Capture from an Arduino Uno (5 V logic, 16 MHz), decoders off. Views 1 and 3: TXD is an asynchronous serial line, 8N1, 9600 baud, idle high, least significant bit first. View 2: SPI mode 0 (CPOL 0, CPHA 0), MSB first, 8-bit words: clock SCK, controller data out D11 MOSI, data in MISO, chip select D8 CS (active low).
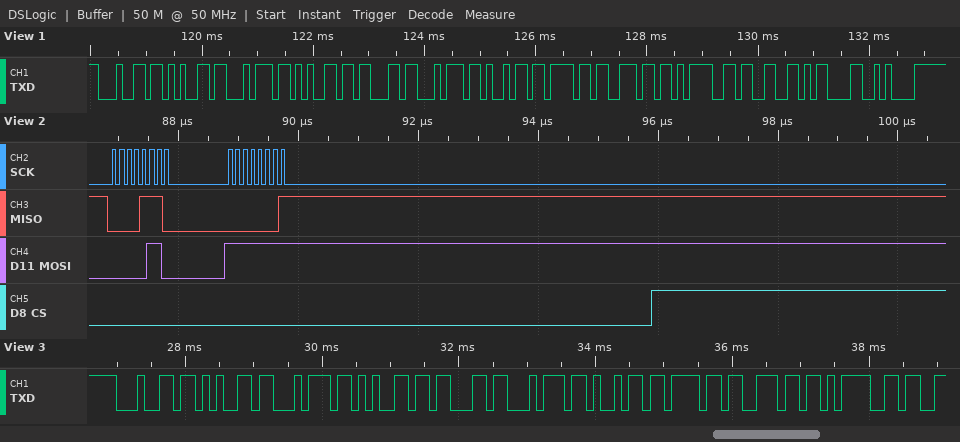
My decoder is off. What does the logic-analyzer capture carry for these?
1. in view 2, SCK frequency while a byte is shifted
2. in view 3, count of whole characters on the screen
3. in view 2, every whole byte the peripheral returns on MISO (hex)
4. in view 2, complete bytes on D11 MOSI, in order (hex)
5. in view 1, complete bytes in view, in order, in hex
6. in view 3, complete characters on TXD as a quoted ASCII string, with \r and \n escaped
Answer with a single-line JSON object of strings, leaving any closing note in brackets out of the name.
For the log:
{"in view 2, SCK frequency while a byte is shifted": "8 MHz", "in view 3, count of whole characters on the screen": "10", "in view 2, every whole byte the peripheral returns on MISO": "0E 01", "in view 2, complete bytes on D11 MOSI, in order": "06 FF", "in view 1, complete bytes in view, in order, in hex": "64 65 74 65 63 74 69 6F 6E 3D 33 0D 0A", "in view 3, complete characters on TXD as a quoted ASCII string, with \\r and \\n escaped": "\"detection=\""}
